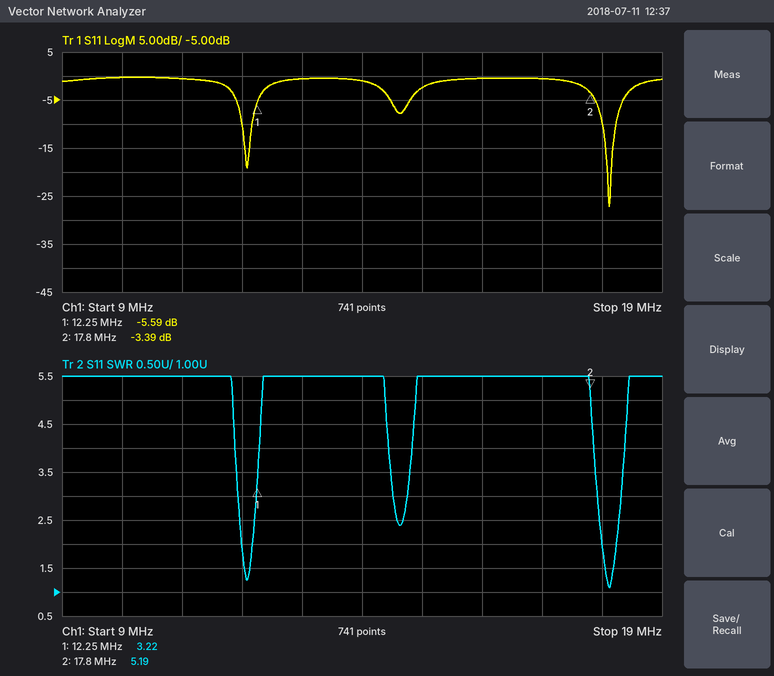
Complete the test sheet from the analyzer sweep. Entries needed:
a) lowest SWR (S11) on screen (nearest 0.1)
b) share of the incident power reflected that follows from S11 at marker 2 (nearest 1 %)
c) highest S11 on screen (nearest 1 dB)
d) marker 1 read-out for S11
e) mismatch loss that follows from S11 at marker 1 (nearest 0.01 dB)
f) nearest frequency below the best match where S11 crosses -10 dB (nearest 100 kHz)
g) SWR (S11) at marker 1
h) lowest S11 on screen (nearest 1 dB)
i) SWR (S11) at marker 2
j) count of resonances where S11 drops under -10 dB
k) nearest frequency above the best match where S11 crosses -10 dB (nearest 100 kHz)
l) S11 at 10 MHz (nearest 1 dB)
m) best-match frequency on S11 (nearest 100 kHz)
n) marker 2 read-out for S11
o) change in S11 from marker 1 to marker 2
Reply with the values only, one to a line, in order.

1.1
46 %
0 dB
-5.59 dB
1.40 dB
18.0 MHz
3.22
-27 dB
5.19
2
18.2 MHz
0 dB
18.1 MHz
-3.39 dB
2.20 dB
